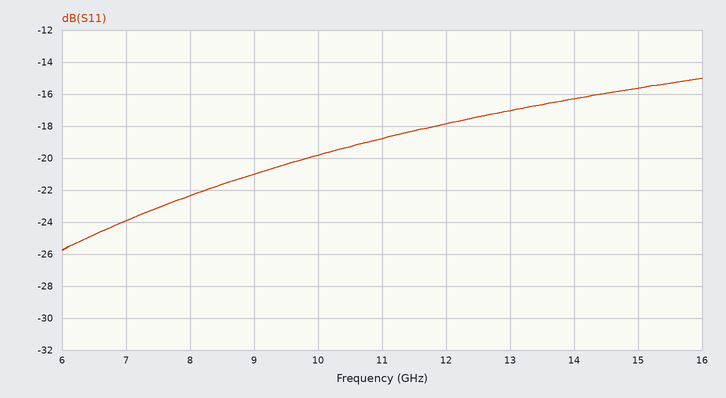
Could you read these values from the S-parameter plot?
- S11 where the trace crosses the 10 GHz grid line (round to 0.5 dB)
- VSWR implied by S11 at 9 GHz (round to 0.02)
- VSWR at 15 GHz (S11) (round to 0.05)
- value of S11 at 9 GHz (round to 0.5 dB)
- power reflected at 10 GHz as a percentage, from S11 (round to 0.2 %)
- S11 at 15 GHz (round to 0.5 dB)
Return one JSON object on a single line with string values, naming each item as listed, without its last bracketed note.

{"S11 where the trace crosses the 10 GHz grid line": "-20.0 dB", "VSWR implied by S11 at 9 GHz": "1.20", "VSWR at 15 GHz (S11)": "1.40", "value of S11 at 9 GHz": "-21.0 dB", "power reflected at 10 GHz as a percentage, from S11": "1.0 %", "S11 at 15 GHz": "-15.5 dB"}
